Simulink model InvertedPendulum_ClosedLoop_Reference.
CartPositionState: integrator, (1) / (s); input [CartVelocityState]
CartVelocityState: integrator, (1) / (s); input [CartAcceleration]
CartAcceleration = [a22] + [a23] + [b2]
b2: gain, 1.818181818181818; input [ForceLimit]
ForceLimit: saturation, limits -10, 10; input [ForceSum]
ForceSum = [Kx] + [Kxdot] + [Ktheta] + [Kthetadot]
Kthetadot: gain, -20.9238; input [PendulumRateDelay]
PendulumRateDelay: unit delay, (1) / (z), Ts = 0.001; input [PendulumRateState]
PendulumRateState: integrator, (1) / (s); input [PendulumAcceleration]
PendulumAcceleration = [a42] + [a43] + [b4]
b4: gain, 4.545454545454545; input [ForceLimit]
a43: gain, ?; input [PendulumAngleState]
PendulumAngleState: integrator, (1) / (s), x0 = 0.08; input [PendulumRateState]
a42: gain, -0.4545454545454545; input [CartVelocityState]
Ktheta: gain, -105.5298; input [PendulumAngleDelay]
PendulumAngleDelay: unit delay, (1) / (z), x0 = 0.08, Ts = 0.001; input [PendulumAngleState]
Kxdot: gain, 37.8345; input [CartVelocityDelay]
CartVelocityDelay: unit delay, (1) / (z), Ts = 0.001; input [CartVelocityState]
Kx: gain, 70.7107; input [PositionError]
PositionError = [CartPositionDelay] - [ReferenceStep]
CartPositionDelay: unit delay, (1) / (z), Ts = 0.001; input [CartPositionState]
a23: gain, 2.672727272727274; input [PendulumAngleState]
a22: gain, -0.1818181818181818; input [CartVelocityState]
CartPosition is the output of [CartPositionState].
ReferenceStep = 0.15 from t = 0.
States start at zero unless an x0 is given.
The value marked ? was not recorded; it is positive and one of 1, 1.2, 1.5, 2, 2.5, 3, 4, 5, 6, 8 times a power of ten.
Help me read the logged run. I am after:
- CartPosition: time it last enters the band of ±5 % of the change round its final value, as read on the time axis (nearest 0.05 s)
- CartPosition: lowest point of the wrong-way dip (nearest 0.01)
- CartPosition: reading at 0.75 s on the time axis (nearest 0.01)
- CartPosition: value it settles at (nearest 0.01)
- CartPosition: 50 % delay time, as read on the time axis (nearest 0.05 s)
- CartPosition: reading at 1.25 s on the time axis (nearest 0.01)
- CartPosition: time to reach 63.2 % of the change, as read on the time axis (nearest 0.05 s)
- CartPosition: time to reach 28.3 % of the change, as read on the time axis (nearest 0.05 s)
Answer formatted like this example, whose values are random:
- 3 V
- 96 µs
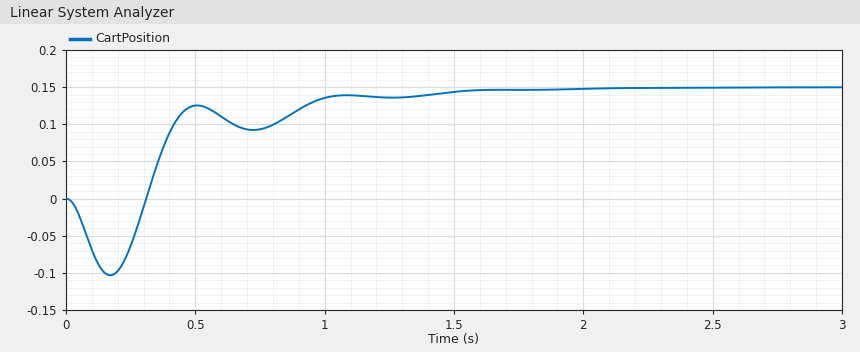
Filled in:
- 1.45 s
- -0.10
- 0.09
- 0.15
- 0.40 s
- 0.14
- 0.40 s
- 0.35 s
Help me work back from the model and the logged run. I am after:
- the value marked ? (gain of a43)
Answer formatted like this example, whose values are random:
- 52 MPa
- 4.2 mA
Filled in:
- 50
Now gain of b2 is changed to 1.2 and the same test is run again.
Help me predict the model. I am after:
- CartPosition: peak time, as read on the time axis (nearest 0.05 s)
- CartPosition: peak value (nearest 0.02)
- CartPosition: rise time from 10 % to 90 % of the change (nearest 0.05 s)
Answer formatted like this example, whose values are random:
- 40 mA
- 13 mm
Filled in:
- 1.00 s
- 0.16
- 0.30 s
